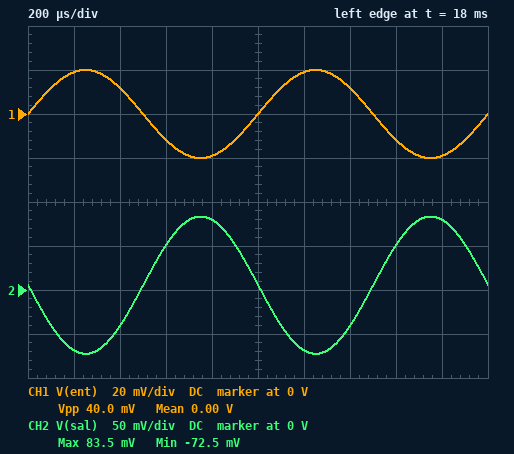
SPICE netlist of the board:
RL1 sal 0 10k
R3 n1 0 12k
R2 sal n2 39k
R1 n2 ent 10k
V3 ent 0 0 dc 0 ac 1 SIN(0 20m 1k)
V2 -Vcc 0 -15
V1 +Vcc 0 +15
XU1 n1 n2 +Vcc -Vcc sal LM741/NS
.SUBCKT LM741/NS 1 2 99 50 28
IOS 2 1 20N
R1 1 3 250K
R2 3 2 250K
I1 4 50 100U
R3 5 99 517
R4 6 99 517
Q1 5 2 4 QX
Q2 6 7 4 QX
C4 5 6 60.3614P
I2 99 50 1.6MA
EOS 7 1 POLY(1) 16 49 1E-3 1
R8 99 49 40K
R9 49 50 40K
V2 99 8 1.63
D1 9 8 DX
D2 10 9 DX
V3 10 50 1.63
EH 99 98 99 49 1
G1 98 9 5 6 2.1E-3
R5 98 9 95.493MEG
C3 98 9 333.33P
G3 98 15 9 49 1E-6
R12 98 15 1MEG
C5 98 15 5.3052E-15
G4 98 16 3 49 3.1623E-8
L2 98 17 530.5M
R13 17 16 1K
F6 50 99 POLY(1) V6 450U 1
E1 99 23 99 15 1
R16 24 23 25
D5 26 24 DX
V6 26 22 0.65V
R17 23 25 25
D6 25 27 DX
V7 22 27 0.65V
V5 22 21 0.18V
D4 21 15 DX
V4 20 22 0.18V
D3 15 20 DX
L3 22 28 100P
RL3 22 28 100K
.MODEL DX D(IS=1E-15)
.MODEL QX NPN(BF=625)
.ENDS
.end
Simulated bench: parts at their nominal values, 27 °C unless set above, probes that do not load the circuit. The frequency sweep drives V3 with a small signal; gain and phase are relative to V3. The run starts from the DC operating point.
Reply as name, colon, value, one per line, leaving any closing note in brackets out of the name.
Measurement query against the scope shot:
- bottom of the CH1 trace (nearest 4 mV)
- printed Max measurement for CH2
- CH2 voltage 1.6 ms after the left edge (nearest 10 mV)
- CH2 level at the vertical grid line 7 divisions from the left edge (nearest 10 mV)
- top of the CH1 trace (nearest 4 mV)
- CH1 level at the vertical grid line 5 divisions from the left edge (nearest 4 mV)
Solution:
bottom of the CH1 trace: -20 mV
printed Max measurement for CH2: 83.5 mV
CH2 voltage 1.6 ms after the left edge: 50 mV
CH2 level at the vertical grid line 7 divisions from the left edge: -40 mV
top of the CH1 trace: 20 mV
CH1 level at the vertical grid line 5 divisions from the left edge: 0 V
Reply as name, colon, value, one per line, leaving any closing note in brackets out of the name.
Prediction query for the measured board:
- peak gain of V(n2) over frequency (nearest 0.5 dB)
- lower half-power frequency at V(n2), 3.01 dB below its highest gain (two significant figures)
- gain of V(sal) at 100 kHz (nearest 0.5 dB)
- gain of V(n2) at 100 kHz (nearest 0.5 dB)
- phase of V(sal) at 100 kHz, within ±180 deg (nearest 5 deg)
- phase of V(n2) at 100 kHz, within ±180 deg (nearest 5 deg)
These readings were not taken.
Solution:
peak gain of V(n2) over frequency: -1.5 dB
lower half-power frequency at V(n2), 3.01 dB below its highest gain: 190 kHz
gain of V(sal) at 100 kHz: 11.0 dB
gain of V(n2) at 100 kHz: -8.5 dB
phase of V(sal) at 100 kHz, within ±180 deg: 150 deg
phase of V(n2) at 100 kHz, within ±180 deg: 65 deg
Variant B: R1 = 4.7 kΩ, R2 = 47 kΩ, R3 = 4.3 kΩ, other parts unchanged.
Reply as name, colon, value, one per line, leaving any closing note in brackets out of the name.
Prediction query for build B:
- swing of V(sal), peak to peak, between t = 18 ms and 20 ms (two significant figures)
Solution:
swing of V(sal), peak to peak, between t = 18 ms and 20 ms: 400 mV
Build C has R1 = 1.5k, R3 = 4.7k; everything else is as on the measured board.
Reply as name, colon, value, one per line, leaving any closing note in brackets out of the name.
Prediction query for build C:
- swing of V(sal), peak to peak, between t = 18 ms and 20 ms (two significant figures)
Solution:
swing of V(sal), peak to peak, between t = 18 ms and 20 ms: 1.0 V
